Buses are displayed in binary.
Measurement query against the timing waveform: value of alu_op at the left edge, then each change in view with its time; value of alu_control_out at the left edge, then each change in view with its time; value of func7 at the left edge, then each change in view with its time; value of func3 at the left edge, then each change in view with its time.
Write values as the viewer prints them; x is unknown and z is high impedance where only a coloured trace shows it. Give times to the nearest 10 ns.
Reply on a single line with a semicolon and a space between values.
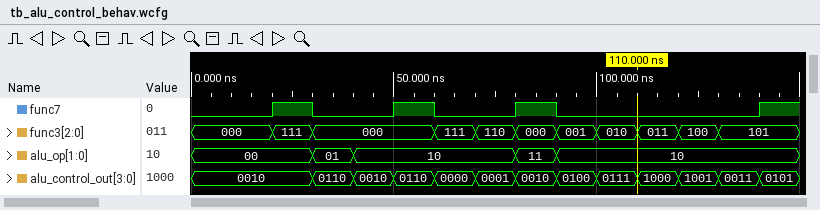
00, 01 at 30 ns, 10 at 40 ns, 11 at 80 ns, 10 at 90 ns; 0010, 0110 at 30 ns, 0010 at 40 ns, 0110 at 50 ns, 0000 at 60 ns, 0001 at 70 ns, 0010 at 80 ns, 0100 at 90 ns, 0111 at 100 ns, 1000 at 110 ns, 1001 at 120 ns, 0011 at 130 ns, 0101 at 140 ns; 0, 1 at 20 ns, 0 at 30 ns, 1 at 50 ns, 0 at 60 ns, 1 at 80 ns, 0 at 90 ns, 1 at 140 ns; 000, 111 at 20 ns, 000 at 30 ns, 111 at 60 ns, 110 at 70 ns, 000 at 80 ns, 001 at 90 ns, 010 at 100 ns, 011 at 110 ns, 100 at 120 ns, 101 at 130 ns
